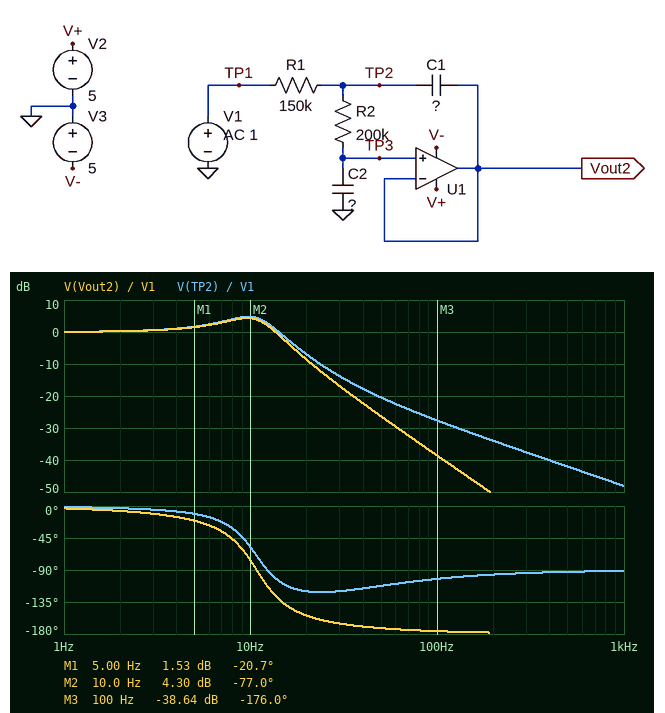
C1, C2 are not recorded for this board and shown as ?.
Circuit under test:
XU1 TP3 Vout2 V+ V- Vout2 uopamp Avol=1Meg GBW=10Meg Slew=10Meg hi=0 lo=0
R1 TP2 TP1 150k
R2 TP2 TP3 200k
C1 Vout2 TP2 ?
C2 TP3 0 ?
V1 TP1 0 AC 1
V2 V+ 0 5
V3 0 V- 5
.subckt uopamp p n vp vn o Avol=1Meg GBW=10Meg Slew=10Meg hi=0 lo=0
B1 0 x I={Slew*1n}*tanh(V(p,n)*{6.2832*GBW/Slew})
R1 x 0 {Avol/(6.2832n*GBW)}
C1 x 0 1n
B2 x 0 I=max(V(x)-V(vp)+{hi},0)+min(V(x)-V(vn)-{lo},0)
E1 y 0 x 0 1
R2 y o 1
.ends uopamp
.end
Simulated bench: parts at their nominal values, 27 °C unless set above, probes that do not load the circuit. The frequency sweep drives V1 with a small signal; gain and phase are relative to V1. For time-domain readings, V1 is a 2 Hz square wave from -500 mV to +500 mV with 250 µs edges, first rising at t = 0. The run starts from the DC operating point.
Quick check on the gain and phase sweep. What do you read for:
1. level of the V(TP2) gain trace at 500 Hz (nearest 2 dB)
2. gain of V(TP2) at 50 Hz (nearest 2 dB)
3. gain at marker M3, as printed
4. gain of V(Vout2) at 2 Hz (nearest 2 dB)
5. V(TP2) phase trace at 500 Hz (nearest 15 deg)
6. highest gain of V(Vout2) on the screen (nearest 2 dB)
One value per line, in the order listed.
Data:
-42 dB
-20 dB
-38.64 dB
0 dB
-90 deg
4 dB
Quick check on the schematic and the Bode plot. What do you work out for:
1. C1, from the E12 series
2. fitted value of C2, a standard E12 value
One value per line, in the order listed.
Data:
270 nF
27 nF
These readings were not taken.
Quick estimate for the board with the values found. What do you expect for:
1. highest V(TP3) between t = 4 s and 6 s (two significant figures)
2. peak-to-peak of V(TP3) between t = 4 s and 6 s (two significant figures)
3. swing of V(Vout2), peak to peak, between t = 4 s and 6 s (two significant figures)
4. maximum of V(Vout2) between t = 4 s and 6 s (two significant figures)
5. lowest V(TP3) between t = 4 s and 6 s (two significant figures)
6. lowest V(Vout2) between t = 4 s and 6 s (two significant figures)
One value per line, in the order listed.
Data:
850 mV
1.7 V
1.7 V
850 mV
-850 mV
-850 mV
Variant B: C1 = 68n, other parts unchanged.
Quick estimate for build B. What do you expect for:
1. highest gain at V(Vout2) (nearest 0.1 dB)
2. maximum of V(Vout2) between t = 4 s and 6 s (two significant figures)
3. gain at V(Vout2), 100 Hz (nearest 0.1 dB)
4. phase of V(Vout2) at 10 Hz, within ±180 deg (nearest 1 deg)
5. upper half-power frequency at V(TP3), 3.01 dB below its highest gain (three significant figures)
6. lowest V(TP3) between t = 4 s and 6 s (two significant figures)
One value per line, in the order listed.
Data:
0.2 dB
580 mV
-26.7 dB
-37 deg
23.2 Hz
-580 mV
